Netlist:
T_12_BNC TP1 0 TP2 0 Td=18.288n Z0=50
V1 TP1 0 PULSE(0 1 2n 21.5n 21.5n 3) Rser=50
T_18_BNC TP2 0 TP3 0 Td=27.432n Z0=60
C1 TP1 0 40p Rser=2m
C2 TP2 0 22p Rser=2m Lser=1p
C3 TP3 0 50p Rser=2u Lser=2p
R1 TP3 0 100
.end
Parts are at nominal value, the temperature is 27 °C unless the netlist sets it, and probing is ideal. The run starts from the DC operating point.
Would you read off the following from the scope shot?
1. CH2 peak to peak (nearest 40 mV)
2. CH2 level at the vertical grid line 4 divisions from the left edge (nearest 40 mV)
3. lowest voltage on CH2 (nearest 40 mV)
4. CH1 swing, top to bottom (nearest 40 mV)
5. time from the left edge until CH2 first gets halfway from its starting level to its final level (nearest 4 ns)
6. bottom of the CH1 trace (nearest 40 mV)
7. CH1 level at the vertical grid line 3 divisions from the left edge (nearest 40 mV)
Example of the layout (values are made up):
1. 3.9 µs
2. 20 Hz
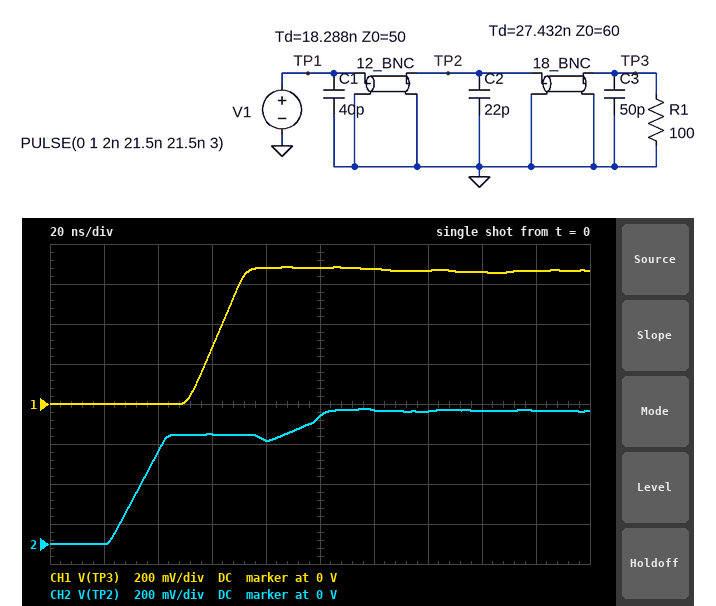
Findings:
1. 680 mV
2. 520 mV
3. 0 V
4. 680 mV
5. 36 ns
6. 0 V
7. 280 mV
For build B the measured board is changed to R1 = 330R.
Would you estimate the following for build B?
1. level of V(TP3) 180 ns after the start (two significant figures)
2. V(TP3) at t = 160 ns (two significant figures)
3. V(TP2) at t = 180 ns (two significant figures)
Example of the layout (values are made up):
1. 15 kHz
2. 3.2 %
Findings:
1. 870 mV
2. 840 mV
3. 860 mV
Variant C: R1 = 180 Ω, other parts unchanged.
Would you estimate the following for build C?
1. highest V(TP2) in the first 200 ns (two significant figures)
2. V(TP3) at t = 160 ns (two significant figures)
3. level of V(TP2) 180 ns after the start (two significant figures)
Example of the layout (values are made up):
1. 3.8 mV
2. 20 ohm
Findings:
1. 800 mV
2. 760 mV
3. 780 mV
